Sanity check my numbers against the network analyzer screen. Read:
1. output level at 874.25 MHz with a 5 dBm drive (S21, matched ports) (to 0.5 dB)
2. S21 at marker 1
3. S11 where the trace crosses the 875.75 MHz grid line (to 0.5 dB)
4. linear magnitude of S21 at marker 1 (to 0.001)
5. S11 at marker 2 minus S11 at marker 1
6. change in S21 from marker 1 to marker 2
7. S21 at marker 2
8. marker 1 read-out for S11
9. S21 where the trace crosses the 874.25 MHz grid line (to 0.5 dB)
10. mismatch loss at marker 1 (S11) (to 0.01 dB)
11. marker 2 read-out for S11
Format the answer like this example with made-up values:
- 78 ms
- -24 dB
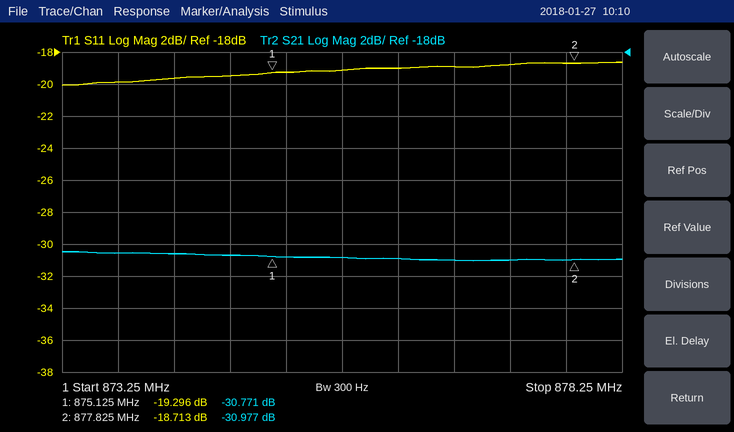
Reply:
- -25.5 dBm
- -30.771 dB
- -19.0 dB
- 0.029
- 0.583 dB
- -0.206 dB
- -30.977 dB
- -19.296 dB
- -30.5 dB
- 0.05 dB
- -18.713 dB
